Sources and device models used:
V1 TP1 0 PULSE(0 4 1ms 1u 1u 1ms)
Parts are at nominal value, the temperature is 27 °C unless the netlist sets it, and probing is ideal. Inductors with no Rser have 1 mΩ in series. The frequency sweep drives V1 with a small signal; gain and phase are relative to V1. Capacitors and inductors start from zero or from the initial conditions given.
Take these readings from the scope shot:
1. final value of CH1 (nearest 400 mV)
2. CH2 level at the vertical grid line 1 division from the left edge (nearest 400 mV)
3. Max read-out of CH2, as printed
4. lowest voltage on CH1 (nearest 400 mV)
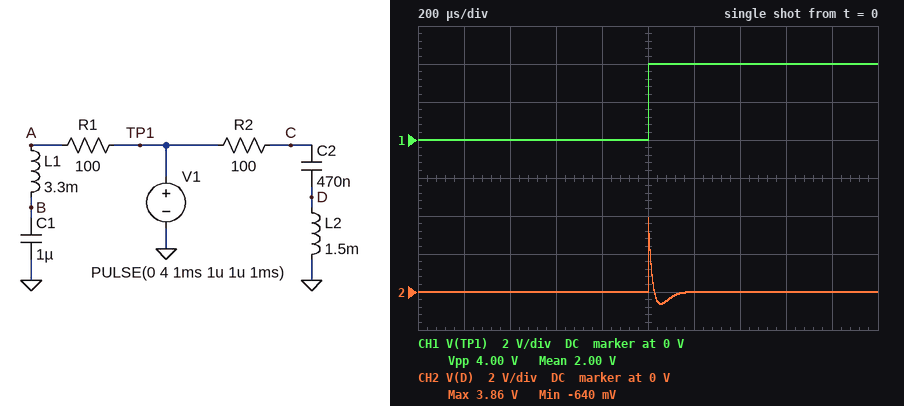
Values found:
4.0 V
0 V
3.86 V
0 V
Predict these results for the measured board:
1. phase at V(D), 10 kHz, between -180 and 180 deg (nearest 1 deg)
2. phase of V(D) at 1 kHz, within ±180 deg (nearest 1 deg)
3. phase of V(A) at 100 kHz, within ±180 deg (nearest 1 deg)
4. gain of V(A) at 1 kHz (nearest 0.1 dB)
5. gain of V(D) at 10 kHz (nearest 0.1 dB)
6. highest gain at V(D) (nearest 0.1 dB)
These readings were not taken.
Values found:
59 deg
163 deg
3 deg
-1.8 dB
-1.9 dB
0 dB
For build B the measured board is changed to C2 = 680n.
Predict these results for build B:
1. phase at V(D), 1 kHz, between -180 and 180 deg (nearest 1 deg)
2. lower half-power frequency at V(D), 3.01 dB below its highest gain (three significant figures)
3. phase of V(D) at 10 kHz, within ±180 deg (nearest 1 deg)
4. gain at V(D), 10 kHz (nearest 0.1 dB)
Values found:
156 deg
8.46 kHz
55 deg
-2.3 dB
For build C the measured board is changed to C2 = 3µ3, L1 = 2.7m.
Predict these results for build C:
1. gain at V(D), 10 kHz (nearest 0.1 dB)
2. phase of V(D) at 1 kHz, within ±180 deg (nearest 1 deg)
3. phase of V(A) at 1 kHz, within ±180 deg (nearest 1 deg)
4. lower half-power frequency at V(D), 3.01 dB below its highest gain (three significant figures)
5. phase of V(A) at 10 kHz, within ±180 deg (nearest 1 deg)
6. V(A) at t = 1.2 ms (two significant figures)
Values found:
-3.1 dB
111 deg
-35 deg
10.1 kHz
33 deg
3.4 V
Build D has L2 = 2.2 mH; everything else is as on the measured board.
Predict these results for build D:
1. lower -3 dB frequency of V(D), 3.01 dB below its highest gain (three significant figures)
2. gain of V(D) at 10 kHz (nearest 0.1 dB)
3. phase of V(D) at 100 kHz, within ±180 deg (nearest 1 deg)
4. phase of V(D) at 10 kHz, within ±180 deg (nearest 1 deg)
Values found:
5.12 kHz
-0.4 dB
4 deg
44 deg
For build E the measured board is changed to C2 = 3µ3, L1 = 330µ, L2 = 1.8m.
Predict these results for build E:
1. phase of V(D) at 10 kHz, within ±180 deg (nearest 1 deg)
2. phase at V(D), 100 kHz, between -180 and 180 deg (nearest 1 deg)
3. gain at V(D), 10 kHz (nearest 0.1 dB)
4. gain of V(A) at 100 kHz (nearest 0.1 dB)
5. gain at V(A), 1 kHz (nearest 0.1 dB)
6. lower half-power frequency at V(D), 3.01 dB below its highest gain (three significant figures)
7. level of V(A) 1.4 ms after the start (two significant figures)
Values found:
43 deg
5 deg
-2.3 dB
-0.9 dB
-1.5 dB
8.36 kHz
3.9 V
